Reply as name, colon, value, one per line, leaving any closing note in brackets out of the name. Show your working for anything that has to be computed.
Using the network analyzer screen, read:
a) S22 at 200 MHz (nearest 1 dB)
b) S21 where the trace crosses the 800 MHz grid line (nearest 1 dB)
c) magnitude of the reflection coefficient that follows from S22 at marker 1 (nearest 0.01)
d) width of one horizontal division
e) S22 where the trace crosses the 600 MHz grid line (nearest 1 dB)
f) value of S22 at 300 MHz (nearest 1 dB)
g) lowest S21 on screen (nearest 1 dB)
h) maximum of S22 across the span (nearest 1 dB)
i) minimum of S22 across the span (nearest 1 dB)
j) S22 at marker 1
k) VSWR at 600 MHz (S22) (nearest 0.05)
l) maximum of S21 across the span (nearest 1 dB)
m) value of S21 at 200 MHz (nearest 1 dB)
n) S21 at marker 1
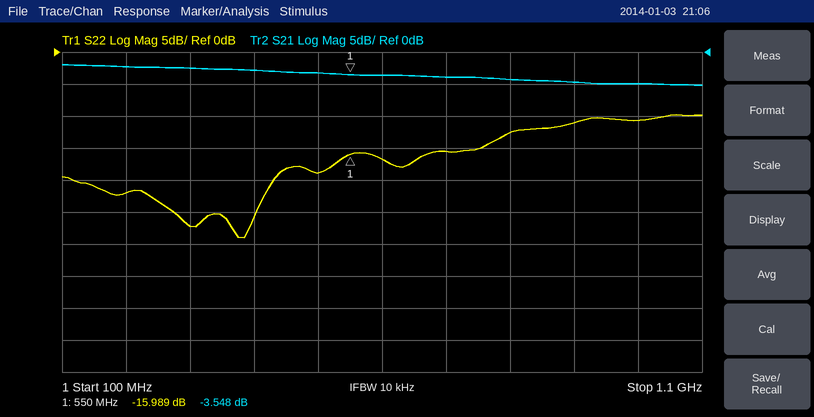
S22 at 200 MHz: -22 dB
S21 where the trace crosses the 800 MHz grid line: -4 dB
magnitude of the reflection coefficient that follows from S22 at marker 1: 10^(-15.989/20) ≈ 0.16
width of one horizontal division: 100 MHz
S22 where the trace crosses the 600 MHz grid line: -17 dB
value of S22 at 300 MHz: -27 dB
lowest S21 on screen: -5 dB
maximum of S22 across the span: -10 dB
minimum of S22 across the span: -29 dB
S22 at marker 1: -15.989 dB
VSWR at 600 MHz (S22): |Γ| = 10^(-17/20) = 0.1413; VSWR = (1 + 0.1413)/(1 − 0.1413) ≈ 1.33, so 1.35 to the nearest 0.05
maximum of S21 across the span: -2 dB
value of S21 at 200 MHz: -2 dB
S21 at marker 1: -3.548 dB
